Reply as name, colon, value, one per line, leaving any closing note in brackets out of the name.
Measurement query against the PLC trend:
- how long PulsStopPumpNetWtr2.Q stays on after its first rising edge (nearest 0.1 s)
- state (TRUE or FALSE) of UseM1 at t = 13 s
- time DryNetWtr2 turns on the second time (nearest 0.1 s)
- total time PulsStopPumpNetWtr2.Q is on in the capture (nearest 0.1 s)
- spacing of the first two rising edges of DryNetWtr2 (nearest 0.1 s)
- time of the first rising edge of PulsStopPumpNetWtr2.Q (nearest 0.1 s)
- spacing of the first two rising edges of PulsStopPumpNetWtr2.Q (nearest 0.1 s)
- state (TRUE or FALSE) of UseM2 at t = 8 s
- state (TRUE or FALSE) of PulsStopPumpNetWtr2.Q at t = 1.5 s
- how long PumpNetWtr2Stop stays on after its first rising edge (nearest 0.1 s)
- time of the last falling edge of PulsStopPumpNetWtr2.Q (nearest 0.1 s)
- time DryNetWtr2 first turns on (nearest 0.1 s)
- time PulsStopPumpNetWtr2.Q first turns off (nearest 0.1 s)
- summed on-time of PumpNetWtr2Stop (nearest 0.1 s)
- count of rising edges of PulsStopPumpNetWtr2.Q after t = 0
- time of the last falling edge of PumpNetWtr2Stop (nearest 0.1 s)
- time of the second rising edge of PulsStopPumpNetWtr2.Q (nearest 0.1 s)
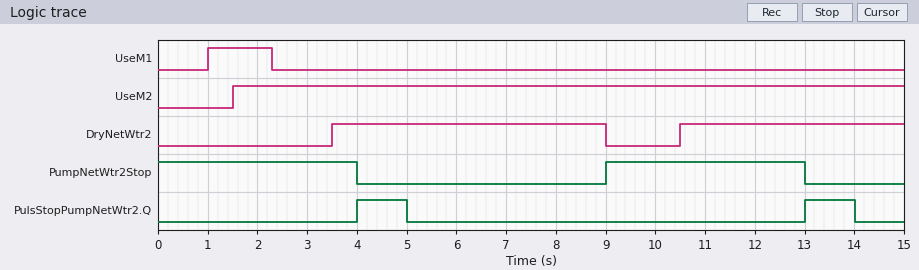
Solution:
how long PulsStopPumpNetWtr2.Q stays on after its first rising edge: 1.0 s
state (TRUE or FALSE) of UseM1 at t = 13 s: FALSE
time DryNetWtr2 turns on the second time: 10.5 s
total time PulsStopPumpNetWtr2.Q is on in the capture: 2.0 s
spacing of the first two rising edges of DryNetWtr2: 7.0 s
time of the first rising edge of PulsStopPumpNetWtr2.Q: 4.0 s
spacing of the first two rising edges of PulsStopPumpNetWtr2.Q: 9.0 s
state (TRUE or FALSE) of UseM2 at t = 8 s: TRUE
state (TRUE or FALSE) of PulsStopPumpNetWtr2.Q at t = 1.5 s: FALSE
how long PumpNetWtr2Stop stays on after its first rising edge: 4.0 s
time of the last falling edge of PulsStopPumpNetWtr2.Q: 14.0 s
time DryNetWtr2 first turns on: 3.5 s
time PulsStopPumpNetWtr2.Q first turns off: 5.0 s
summed on-time of PumpNetWtr2Stop: 8.0 s
count of rising edges of PulsStopPumpNetWtr2.Q after t = 0: 2
time of the last falling edge of PumpNetWtr2Stop: 13.0 s
time of the second rising edge of PulsStopPumpNetWtr2.Q: 13.0 s
